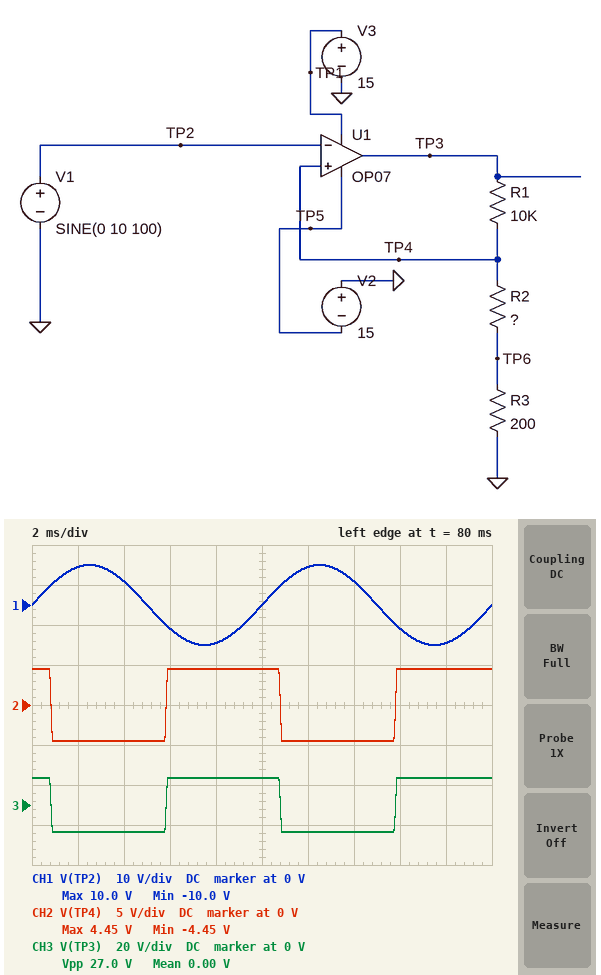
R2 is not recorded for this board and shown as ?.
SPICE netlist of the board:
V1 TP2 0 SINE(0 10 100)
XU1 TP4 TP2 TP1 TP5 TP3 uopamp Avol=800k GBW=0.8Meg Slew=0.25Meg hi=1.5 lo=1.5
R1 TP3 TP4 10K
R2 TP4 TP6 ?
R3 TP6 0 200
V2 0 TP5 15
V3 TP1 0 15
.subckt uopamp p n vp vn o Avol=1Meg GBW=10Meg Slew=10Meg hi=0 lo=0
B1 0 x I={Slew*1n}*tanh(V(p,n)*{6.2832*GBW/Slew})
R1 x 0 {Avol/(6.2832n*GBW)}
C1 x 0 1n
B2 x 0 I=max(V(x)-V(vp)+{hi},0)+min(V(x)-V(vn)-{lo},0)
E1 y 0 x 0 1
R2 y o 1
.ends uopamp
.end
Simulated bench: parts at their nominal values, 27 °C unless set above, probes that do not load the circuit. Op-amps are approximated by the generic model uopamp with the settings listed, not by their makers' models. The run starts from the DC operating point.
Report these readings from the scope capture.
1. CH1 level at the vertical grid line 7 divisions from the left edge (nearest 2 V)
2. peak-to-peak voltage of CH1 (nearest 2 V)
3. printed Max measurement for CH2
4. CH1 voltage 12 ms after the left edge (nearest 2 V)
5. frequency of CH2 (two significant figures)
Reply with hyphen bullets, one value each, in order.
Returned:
- 6 V
- 20 V
- 4.45 V
- 10 V
- 100 Hz
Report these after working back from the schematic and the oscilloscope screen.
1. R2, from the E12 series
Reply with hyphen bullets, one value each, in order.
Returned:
- 4.7 kΩ
